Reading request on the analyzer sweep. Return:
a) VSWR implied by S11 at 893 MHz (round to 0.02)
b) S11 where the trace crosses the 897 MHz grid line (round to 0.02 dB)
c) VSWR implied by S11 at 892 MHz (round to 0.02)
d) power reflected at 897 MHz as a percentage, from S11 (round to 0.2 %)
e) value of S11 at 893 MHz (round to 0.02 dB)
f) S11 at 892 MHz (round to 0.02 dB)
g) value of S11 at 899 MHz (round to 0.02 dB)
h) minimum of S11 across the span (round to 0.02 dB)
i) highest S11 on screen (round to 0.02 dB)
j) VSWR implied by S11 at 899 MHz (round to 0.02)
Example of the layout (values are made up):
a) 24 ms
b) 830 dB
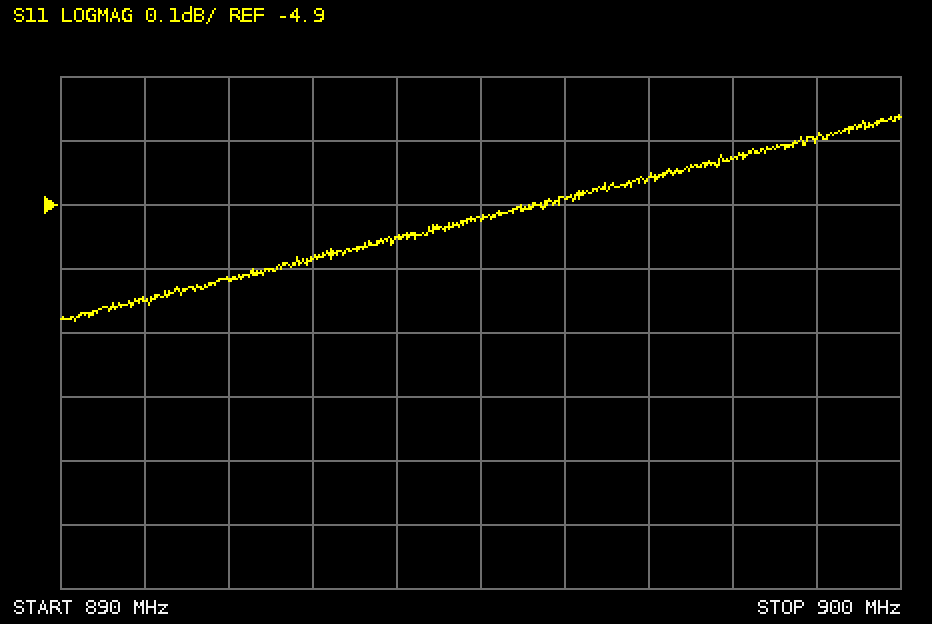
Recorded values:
a) 3.58
b) -4.86 dB
c) 3.56
d) 32.6 %
e) -4.98 dB
f) -5.02 dB
g) -4.80 dB
h) -5.08 dB
i) -4.76 dB
j) 3.72
